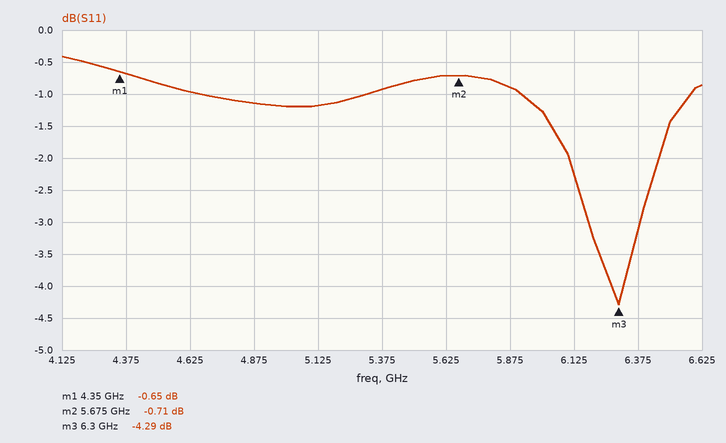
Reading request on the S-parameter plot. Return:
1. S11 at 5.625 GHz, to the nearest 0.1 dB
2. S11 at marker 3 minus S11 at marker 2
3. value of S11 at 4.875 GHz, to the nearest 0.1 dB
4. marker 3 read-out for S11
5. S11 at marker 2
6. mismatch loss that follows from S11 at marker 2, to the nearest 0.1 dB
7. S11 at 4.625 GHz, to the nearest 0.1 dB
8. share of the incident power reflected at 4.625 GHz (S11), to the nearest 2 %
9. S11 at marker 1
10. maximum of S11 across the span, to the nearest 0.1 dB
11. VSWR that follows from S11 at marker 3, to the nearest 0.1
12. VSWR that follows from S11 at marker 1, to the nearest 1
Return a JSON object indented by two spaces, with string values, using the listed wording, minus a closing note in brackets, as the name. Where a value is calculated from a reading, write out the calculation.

{
  "S11 at 5.625 GHz, to the nearest 0.1 dB": "-0.7 dB",
  "S11 at marker 3 minus S11 at marker 2": "-4.29 − (-0.71) = -3.58 dB",
  "value of S11 at 4.875 GHz, to the nearest 0.1 dB": "-1.1 dB",
  "marker 3 read-out for S11": "-4.29 dB",
  "S11 at marker 2": "-0.71 dB",
  "mismatch loss that follows from S11 at marker 2, to the nearest 0.1 dB": "−10 log10(1 − 10^(-0.71/10)) ≈ 8.2 dB",
  "S11 at 4.625 GHz, to the nearest 0.1 dB": "-1.0 dB",
  "share of the incident power reflected at 4.625 GHz (S11), to the nearest 2 %": "10^(-1/10) ≈ 79.4 %, so 80 % to the nearest 2 %",
  "S11 at marker 1": "-0.65 dB",
  "maximum of S11 across the span, to the nearest 0.1 dB": "-0.4 dB",
  "VSWR that follows from S11 at marker 3, to the nearest 0.1": "(1 + 0.6102)/(1 − 0.6102) ≈ 4.1",
  "VSWR that follows from S11 at marker 1, to the nearest 1": "(1 + 0.9279)/(1 − 0.9279) ≈ 27"
}
